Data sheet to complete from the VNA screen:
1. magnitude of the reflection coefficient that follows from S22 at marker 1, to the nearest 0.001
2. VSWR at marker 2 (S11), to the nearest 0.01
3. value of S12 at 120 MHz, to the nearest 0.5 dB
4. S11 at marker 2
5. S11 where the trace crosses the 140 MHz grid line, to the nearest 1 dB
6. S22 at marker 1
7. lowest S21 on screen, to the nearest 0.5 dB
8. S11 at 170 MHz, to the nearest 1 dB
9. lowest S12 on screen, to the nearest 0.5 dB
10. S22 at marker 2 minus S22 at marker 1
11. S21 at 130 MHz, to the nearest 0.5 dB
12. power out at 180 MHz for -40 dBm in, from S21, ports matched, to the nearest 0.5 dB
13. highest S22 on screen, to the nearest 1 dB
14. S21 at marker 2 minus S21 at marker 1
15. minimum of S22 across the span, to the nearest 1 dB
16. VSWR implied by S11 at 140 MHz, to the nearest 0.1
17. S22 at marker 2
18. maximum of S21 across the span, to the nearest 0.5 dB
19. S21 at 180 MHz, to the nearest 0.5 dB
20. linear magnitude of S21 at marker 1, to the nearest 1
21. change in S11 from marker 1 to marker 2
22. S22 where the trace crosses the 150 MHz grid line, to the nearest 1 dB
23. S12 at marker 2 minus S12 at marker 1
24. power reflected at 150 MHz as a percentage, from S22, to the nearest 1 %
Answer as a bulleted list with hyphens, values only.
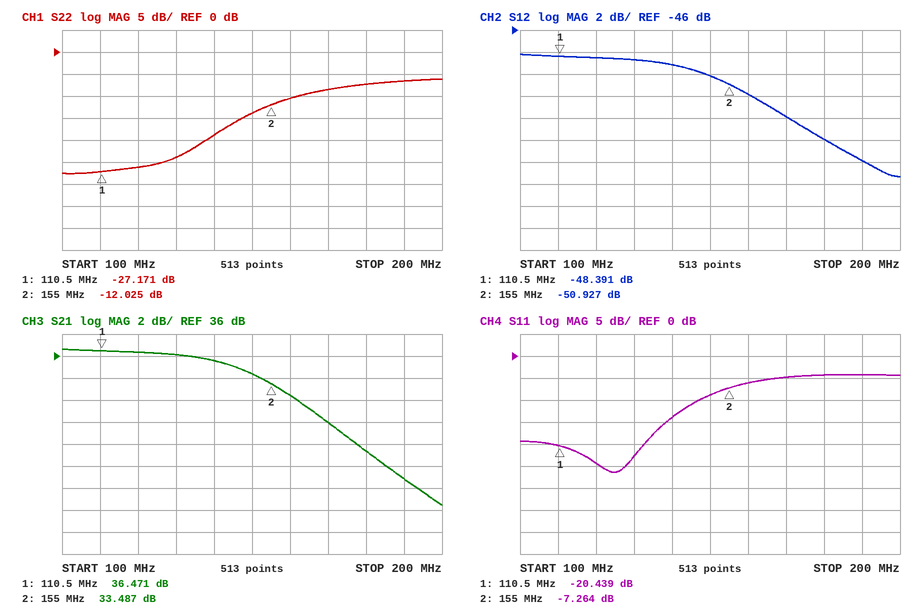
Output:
- 0.044
- 2.53
- -48.5 dB
- -7.264 dB
- -14 dB
- -27.171 dB
- 22.5 dB
- -5 dB
- -59.5 dB
- 15.146 dB
- 36.0 dB
- -12.5 dBm
- -6 dB
- -2.984 dB
- -28 dB
- 1.5
- -12.025 dB
- 36.5 dB
- 27.5 dB
- 67
- 13.175 dB
- -14 dB
- -2.536 dB
- 4 %
